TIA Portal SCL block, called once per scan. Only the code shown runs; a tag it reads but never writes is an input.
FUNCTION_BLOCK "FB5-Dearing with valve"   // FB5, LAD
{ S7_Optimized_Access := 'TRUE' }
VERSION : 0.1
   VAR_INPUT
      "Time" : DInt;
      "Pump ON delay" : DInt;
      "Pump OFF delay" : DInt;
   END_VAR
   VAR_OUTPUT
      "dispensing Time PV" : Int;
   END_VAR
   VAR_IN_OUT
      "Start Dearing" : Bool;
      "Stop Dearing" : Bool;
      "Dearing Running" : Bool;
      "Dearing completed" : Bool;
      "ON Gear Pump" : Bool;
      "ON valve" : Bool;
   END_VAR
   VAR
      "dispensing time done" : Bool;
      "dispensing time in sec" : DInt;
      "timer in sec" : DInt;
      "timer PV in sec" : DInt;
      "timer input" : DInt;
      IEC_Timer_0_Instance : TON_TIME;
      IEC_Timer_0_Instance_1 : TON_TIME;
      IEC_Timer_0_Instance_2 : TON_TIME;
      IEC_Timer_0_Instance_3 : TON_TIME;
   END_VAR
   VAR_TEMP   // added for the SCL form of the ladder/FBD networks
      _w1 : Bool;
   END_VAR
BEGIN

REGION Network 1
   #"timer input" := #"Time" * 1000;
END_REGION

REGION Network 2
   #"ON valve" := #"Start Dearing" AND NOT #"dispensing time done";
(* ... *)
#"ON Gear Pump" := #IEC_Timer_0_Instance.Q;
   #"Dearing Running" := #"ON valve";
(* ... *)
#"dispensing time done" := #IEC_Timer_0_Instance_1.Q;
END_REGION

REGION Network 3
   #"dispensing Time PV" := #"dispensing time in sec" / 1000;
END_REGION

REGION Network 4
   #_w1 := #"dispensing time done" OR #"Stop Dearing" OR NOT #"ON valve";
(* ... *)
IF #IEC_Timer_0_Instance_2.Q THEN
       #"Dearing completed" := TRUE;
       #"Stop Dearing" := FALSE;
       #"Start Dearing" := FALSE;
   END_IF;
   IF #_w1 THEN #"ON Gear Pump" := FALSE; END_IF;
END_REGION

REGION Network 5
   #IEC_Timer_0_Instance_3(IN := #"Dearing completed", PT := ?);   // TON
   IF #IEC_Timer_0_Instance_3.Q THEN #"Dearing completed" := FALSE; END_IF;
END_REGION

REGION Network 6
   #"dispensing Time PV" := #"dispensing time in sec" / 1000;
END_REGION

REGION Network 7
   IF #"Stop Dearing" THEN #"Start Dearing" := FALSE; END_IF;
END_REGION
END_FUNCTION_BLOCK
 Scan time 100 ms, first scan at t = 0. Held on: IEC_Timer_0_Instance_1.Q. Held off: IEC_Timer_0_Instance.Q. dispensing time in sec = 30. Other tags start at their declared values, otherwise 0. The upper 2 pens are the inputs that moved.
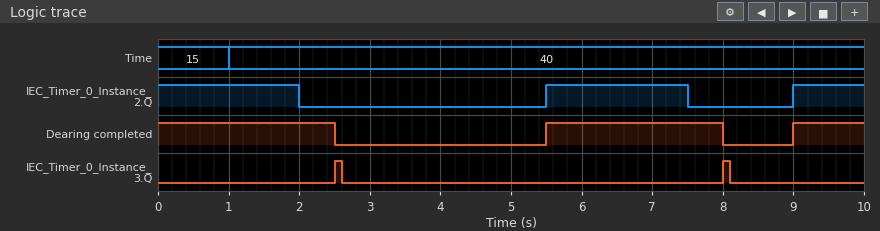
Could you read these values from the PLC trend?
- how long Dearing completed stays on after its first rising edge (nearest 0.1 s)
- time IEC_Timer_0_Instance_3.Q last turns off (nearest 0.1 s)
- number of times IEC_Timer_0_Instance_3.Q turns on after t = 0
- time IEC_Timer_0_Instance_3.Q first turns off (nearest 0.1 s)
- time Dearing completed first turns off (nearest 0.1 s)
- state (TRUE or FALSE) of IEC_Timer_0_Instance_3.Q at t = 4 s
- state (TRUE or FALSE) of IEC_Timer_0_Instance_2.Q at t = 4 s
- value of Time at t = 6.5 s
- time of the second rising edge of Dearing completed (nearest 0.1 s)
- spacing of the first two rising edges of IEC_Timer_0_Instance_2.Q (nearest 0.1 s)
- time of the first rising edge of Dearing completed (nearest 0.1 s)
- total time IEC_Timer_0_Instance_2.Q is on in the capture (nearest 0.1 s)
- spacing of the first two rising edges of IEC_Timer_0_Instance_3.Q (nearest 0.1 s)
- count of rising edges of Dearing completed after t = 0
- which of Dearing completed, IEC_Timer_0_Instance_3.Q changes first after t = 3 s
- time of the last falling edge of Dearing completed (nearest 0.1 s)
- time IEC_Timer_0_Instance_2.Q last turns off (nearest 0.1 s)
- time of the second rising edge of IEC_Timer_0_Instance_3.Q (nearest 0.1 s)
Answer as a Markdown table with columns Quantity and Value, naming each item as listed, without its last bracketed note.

| Quantity | Value |
|---|---|
| how long Dearing completed stays on after its first rising edge | 2.5 s |
| time IEC_Timer_0_Instance_3.Q last turns off | 8.1 s |
| number of times IEC_Timer_0_Instance_3.Q turns on after t = 0 | 2 |
| time IEC_Timer_0_Instance_3.Q first turns off | 2.6 s |
| time Dearing completed first turns off | 2.5 s |
| state (TRUE or FALSE) of IEC_Timer_0_Instance_3.Q at t = 4 s | FALSE |
| state (TRUE or FALSE) of IEC_Timer_0_Instance_2.Q at t = 4 s | FALSE |
| value of Time at t = 6.5 s | 40 |
| time of the second rising edge of Dearing completed | 9.0 s |
| spacing of the first two rising edges of IEC_Timer_0_Instance_2.Q | 3.5 s |
| time of the first rising edge of Dearing completed | 5.5 s |
| total time IEC_Timer_0_Instance_2.Q is on in the capture | 5.0 s |
| spacing of the first two rising edges of IEC_Timer_0_Instance_3.Q | 5.5 s |
| count of rising edges of Dearing completed after t = 0 | 2 |
| which of Dearing completed, IEC_Timer_0_Instance_3.Q changes first after t = 3 s | Dearing completed |
| time of the last falling edge of Dearing completed | 8.0 s |
| time IEC_Timer_0_Instance_2.Q last turns off | 7.5 s |
| time of the second rising edge of IEC_Timer_0_Instance_3.Q | 8.0 s |
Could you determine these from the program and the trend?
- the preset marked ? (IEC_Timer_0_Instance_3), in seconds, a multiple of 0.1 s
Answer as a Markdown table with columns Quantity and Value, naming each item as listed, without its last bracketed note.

| Quantity | Value |
|---|---|
| the preset marked ? (IEC_Timer_0_Instance_3), in seconds, a multiple of 0.1 s | 2.5 s |
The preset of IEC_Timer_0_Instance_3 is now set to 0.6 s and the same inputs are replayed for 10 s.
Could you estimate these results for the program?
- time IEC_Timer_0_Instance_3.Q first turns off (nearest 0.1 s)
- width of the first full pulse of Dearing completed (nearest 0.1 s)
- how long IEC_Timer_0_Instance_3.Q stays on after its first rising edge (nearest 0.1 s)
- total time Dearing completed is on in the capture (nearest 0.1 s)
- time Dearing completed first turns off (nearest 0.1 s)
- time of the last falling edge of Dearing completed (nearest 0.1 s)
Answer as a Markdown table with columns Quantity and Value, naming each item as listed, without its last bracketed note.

| Quantity | Value |
|---|---|
| time IEC_Timer_0_Instance_3.Q first turns off | 2.0 s |
| width of the first full pulse of Dearing completed | 0.6 s |
| how long IEC_Timer_0_Instance_3.Q stays on after its first rising edge | 1.4 s |
| total time Dearing completed is on in the capture | 1.8 s |
| time Dearing completed first turns off | 0.6 s |
| time of the last falling edge of Dearing completed | 9.6 s |
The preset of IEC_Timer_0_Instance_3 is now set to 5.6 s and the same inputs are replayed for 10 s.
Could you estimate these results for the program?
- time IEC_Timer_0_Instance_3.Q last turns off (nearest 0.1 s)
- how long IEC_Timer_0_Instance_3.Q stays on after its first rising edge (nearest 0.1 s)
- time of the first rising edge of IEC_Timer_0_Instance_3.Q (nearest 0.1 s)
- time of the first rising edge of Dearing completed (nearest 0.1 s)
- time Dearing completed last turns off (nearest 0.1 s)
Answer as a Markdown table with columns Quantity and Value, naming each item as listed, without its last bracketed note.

| Quantity | Value |
|---|---|
| time IEC_Timer_0_Instance_3.Q last turns off | 7.5 s |
| how long IEC_Timer_0_Instance_3.Q stays on after its first rising edge | 1.9 s |
| time of the first rising edge of IEC_Timer_0_Instance_3.Q | 5.6 s |
| time of the first rising edge of Dearing completed | 9.0 s |
| time Dearing completed last turns off | 5.6 s |
